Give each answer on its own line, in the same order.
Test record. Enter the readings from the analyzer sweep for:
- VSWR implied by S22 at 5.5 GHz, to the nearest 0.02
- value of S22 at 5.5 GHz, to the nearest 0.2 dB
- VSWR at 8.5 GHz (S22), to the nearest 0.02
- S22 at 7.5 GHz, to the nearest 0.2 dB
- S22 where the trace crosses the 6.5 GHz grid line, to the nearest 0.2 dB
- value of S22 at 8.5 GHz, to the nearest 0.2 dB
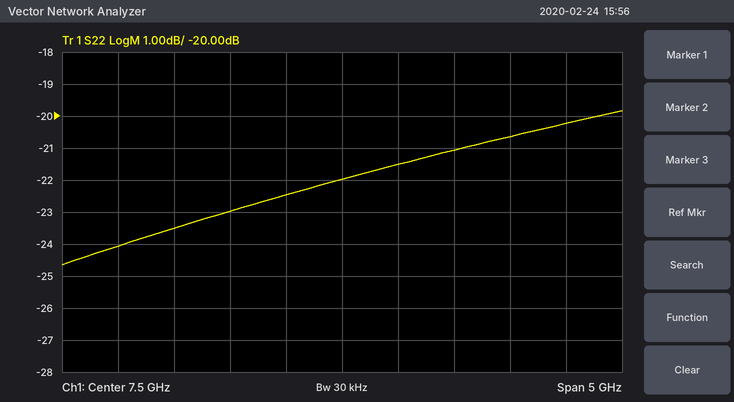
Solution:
1.14
-24.0 dB
1.20
-22.0 dB
-23.0 dB
-21.0 dB
